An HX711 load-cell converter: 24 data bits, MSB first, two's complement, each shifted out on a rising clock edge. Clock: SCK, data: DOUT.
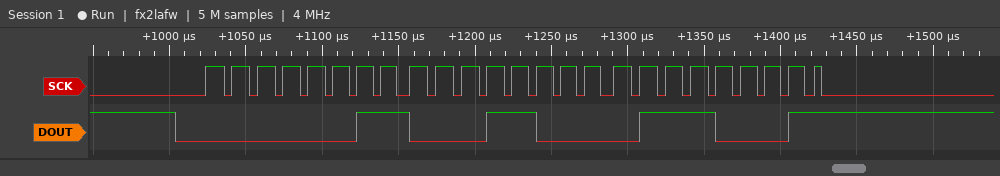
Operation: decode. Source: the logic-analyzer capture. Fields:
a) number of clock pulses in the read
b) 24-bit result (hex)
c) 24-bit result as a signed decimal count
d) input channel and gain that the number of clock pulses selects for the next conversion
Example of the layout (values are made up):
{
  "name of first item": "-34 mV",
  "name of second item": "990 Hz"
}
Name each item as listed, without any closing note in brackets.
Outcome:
{
  "number of clock pulses in the read": "25",
  "24-bit result": "0x031871",
  "24-bit result as a signed decimal count": "202865",
  "input channel and gain that the number of clock pulses selects for the next conversion": "channel A, gain 128"
}
